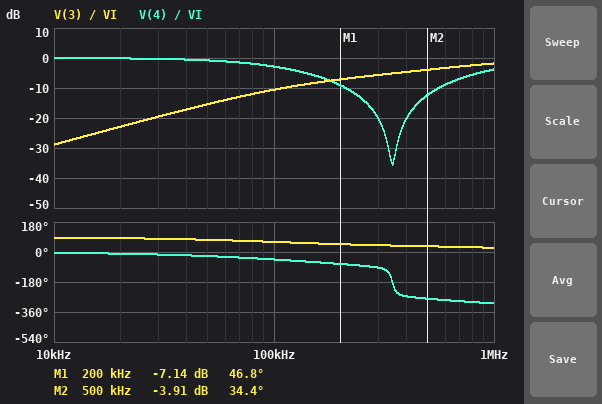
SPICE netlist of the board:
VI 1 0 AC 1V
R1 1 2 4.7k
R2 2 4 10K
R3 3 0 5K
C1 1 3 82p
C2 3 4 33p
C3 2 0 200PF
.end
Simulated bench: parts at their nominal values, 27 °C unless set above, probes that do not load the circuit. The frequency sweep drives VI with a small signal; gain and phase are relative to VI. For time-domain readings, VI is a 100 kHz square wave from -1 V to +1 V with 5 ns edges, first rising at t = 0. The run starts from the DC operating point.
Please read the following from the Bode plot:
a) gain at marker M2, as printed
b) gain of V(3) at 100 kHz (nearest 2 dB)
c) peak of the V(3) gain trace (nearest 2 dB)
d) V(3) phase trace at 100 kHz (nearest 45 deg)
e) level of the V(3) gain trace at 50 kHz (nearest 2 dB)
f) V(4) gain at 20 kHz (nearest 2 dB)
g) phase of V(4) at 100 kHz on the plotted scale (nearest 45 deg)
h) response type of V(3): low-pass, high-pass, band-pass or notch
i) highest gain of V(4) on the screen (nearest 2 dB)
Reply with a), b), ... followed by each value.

a) -3.91 dB
b) -10 dB
c) -2 dB
d) 45 deg
e) -16 dB
f) 0 dB
g) -45 deg
h) high-pass
i) 0 dB
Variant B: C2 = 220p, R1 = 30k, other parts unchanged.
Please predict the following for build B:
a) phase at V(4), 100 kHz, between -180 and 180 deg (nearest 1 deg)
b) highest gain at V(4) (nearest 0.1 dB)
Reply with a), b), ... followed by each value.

a) 87 deg
b) 0 dB
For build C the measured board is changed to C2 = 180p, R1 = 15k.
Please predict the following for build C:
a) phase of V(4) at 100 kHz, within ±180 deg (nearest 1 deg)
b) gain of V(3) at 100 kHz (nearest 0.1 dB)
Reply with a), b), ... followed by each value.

a) -79 deg
b) -13.7 dB
